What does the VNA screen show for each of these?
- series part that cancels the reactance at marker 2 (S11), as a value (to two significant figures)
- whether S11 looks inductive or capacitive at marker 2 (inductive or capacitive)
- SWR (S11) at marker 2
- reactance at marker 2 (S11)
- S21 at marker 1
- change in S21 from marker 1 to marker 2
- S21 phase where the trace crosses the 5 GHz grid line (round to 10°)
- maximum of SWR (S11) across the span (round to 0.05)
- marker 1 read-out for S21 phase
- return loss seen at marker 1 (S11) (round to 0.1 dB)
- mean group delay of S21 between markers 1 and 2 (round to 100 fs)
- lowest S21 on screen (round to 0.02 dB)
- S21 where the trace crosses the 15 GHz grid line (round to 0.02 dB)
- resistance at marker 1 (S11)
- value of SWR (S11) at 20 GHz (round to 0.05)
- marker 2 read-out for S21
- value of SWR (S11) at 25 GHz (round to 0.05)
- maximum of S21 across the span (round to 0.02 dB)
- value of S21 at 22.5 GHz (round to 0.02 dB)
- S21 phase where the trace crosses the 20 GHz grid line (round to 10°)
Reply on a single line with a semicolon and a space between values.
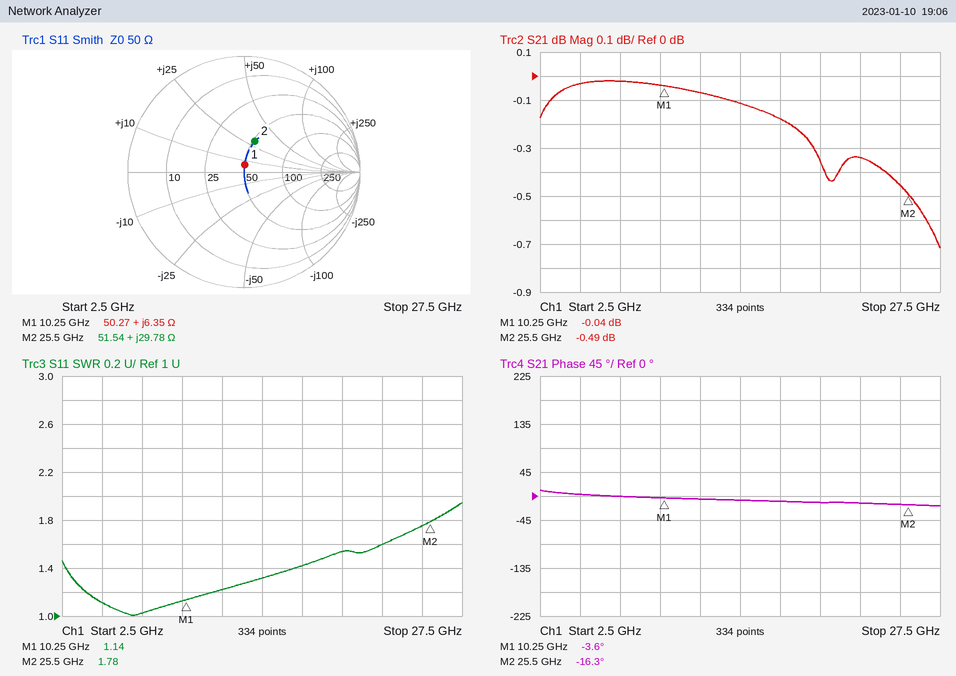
210 fF; inductive; 1.78; +29.78 Ω; -0.04 dB; -0.45 dB; 0°; 1.95; -3.6°; 24.0 dB; 2.3 ps; -0.72 dB; -0.12 dB; 50.27 Ω; 1.55; -0.49 dB; 1.75; -0.02 dB; -0.34 dB; -10°
